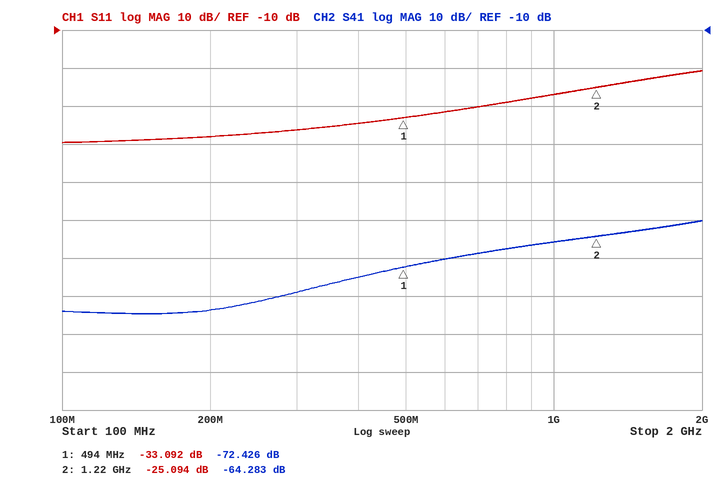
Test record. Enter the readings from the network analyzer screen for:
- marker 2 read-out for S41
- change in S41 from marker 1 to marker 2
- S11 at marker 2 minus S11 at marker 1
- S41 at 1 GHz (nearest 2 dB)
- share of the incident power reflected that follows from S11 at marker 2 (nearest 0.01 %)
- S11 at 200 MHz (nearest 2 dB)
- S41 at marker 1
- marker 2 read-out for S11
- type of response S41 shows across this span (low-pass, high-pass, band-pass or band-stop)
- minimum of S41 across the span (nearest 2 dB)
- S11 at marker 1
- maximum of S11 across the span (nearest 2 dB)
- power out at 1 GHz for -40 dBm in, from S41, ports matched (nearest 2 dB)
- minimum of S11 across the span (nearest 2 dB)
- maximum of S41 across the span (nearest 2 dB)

-64.283 dB
8.143 dB
7.998 dB
-66 dB
0.31 %
-38 dB
-72.426 dB
-25.094 dB
high-pass
-84 dB
-33.092 dB
-20 dB
-106 dBm
-40 dB
-60 dB
